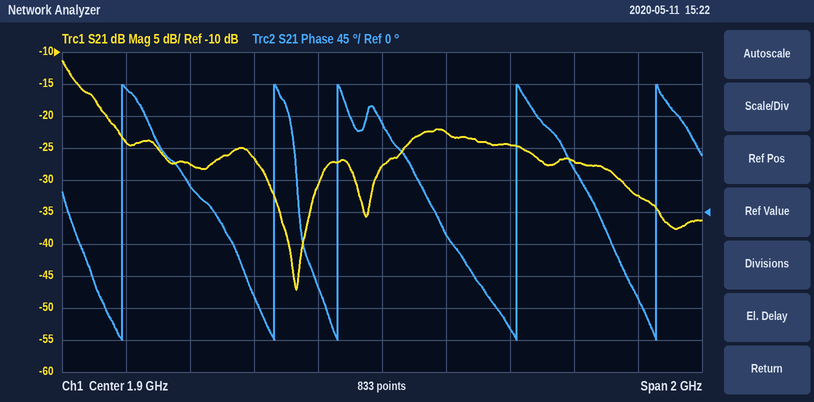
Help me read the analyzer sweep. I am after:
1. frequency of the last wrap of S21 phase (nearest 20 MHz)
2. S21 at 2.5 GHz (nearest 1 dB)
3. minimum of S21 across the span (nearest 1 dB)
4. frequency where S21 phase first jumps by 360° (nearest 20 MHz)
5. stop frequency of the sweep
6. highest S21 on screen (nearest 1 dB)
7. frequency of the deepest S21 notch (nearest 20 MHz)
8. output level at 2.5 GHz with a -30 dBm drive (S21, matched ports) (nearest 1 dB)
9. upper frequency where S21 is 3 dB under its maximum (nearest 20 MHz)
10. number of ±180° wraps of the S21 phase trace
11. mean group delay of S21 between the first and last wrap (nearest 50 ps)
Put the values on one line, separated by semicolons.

2.76 GHz; -27 dB; -47 dB; 1.08 GHz; 2.9 GHz; -11 dB; 1.64 GHz; -57 dBm; 940 MHz; 5; 2.40 ns
